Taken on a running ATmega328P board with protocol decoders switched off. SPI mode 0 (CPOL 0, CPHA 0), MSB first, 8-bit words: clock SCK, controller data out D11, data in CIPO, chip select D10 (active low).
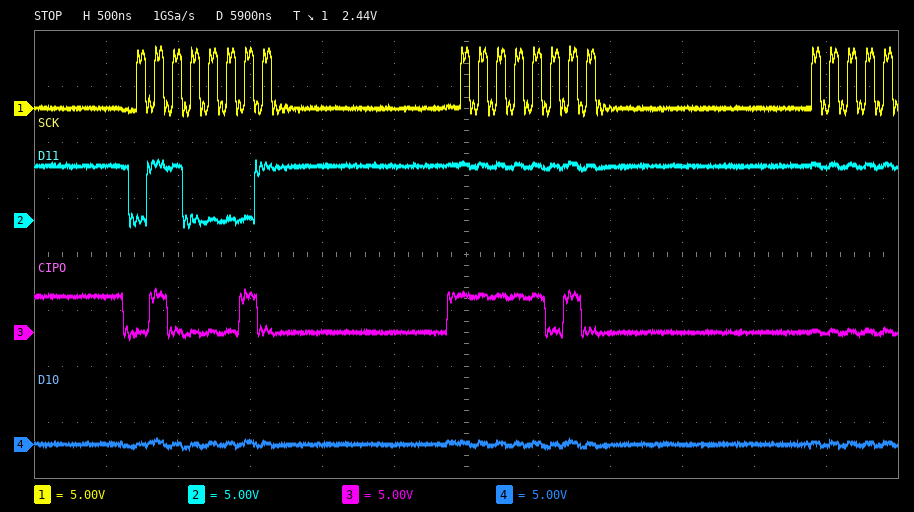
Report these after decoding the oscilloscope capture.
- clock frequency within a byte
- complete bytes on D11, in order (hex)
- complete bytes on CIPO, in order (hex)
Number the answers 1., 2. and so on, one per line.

1. 8 MHz
2. 61 FF
3. 42 FA
